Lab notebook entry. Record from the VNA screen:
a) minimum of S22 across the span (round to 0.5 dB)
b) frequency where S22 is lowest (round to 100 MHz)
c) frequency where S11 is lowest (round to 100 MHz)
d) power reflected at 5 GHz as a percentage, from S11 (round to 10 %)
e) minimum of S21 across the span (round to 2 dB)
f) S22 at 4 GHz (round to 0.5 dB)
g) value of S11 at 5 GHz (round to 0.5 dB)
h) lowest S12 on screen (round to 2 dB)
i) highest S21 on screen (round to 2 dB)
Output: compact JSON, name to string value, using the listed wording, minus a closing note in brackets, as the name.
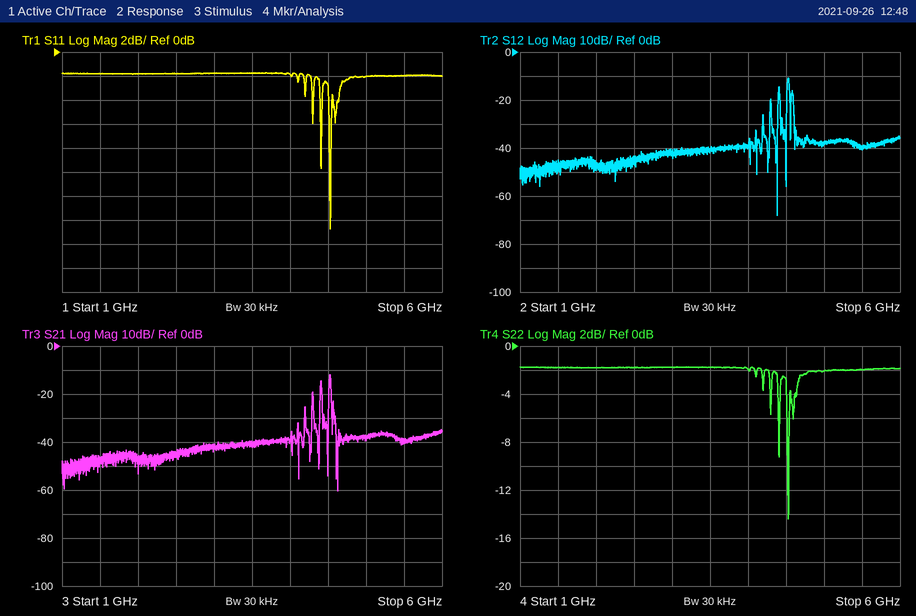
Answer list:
{"minimum of S22 across the span": "-14.5 dB", "frequency where S22 is lowest": "4.5 GHz", "frequency where S11 is lowest": "4.5 GHz", "power reflected at 5 GHz as a percentage, from S11": "60 %", "minimum of S21 across the span": "-60 dB", "S22 at 4 GHz": "-2.0 dB", "value of S11 at 5 GHz": "-2.0 dB", "lowest S12 on screen": "-68 dB", "highest S21 on screen": "-12 dB"}
